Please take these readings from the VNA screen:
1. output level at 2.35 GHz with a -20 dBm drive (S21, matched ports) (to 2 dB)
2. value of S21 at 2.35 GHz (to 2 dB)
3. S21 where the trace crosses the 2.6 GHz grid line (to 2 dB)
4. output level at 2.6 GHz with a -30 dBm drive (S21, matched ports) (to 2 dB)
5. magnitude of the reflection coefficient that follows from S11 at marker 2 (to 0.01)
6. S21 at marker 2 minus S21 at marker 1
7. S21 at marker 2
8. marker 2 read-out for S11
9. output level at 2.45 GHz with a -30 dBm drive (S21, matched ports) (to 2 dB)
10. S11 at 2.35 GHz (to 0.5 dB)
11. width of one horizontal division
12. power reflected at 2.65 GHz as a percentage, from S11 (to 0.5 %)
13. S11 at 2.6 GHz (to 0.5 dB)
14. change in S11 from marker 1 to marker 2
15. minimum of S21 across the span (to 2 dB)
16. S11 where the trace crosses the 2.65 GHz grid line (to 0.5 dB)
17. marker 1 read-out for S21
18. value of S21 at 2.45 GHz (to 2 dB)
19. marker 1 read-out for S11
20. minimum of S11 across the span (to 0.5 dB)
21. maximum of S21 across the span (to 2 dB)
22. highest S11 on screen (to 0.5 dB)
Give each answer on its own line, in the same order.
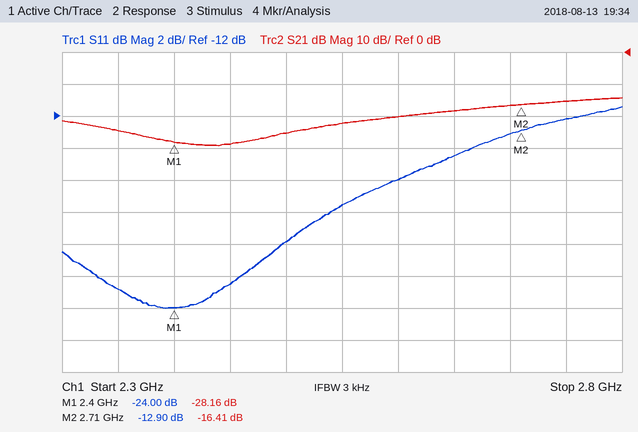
-44 dBm
-24 dB
-20 dB
-50 dBm
0.23
11.75 dB
-16.41 dB
-12.90 dB
-58 dBm
-23.0 dB
50 MHz
3.5 %
-16.0 dB
11.10 dB
-30 dB
-14.5 dB
-28.16 dB
-28 dB
-24.00 dB
-24.0 dB
-14 dB
-11.5 dB
